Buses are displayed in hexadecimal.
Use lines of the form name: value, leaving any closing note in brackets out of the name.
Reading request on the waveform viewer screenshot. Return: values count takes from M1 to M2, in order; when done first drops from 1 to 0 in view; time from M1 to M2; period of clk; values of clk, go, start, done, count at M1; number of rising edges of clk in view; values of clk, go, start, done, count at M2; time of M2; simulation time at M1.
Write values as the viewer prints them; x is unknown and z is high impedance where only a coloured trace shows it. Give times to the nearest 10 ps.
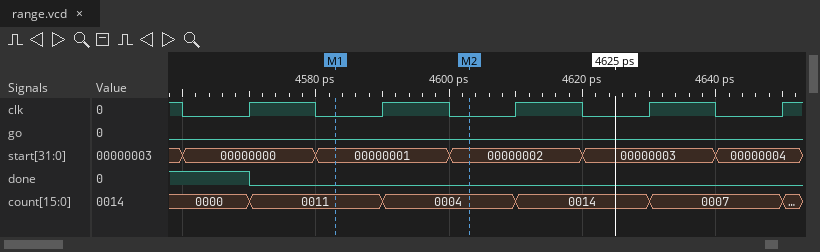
values count takes from M1 to M2, in order: 0011, 0004
when done first drops from 1 to 0 in view: 4570 ps
time from M1 to M2: 20 ps
period of clk: 20 ps
values of clk, go, start, done, count at M1: clk=0, go=0, start=00000001, done=0, count=0011
number of rising edges of clk in view: 5
values of clk, go, start, done, count at M2: clk=0, go=0, start=00000002, done=0, count=0004
time of M2: 4600 ps
simulation time at M1: 4580 ps
